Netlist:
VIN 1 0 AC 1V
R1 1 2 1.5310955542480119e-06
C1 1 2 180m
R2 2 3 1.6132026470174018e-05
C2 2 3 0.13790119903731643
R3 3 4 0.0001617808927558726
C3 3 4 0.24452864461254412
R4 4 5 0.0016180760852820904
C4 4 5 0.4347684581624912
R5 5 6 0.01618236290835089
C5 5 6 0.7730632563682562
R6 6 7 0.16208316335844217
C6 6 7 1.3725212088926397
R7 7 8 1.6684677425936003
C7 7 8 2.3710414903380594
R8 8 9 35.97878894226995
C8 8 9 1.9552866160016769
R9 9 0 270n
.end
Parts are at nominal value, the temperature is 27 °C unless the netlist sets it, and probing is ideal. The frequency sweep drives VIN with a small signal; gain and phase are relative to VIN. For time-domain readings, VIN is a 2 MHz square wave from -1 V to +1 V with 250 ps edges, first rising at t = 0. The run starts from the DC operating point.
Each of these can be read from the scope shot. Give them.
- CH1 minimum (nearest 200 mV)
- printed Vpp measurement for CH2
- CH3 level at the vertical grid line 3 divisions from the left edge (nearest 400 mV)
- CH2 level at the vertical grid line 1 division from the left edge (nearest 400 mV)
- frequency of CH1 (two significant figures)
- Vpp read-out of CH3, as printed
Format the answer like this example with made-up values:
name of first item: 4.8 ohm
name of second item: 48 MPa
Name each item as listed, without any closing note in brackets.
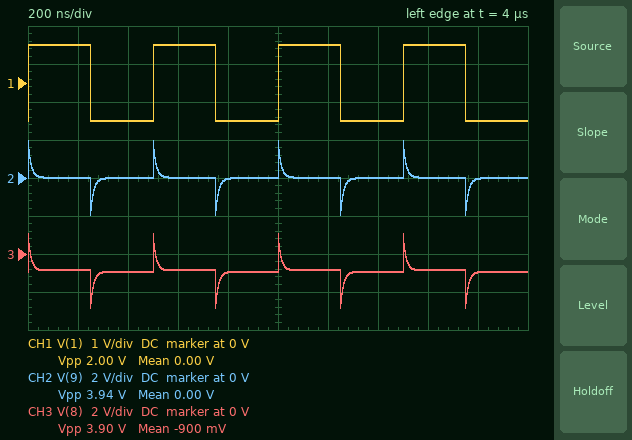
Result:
CH1 minimum: -1.0 V
printed Vpp measurement for CH2: 3.94 V
CH3 level at the vertical grid line 3 divisions from the left edge: -800 mV
CH2 level at the vertical grid line 1 division from the left edge: 0 V
frequency of CH1: 2.0 MHz
Vpp read-out of CH3, as printed: 3.90 V
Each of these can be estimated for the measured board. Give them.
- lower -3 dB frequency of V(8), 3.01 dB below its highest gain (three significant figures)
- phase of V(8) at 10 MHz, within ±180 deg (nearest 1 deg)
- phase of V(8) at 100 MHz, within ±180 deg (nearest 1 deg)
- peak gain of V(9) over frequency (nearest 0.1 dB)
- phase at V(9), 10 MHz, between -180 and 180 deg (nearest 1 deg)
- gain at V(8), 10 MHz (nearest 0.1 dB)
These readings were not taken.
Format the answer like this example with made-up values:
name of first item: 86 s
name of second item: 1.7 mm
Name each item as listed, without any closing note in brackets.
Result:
lower -3 dB frequency of V(8), 3.01 dB below its highest gain: 13.2 MHz
phase of V(8) at 10 MHz, within ±180 deg: 50 deg
phase of V(8) at 100 MHz, within ±180 deg: 7 deg
peak gain of V(9) over frequency: 0 dB
phase at V(9), 10 MHz, between -180 and 180 deg: 52 deg
gain at V(8), 10 MHz: -4.4 dB
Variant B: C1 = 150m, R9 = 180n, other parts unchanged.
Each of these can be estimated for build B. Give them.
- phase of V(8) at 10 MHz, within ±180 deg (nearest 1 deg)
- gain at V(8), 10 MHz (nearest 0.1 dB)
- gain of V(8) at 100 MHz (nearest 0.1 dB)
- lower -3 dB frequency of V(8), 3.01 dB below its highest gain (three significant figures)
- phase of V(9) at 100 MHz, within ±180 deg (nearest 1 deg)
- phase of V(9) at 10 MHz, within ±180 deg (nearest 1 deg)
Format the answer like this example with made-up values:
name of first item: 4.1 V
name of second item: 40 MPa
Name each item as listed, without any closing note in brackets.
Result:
phase of V(8) at 10 MHz, within ±180 deg: 60 deg
gain at V(8), 10 MHz: -7.2 dB
gain of V(8) at 100 MHz: -0.2 dB
lower -3 dB frequency of V(8), 3.01 dB below its highest gain: 20.8 MHz
phase of V(9) at 100 MHz, within ±180 deg: 12 deg
phase of V(9) at 10 MHz, within ±180 deg: 63 deg
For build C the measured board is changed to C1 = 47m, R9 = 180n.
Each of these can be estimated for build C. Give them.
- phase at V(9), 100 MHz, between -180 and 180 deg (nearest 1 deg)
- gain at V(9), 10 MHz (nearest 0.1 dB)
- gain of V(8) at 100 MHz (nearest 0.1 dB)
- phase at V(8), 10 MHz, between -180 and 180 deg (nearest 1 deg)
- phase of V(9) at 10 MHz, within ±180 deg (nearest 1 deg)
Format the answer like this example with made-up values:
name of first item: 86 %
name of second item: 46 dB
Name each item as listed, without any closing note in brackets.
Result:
phase at V(9), 100 MHz, between -180 and 180 deg: 18 deg
gain at V(9), 10 MHz: -11.0 dB
gain of V(8) at 100 MHz: -0.5 dB
phase at V(8), 10 MHz, between -180 and 180 deg: 64 deg
phase of V(9) at 10 MHz, within ±180 deg: 67 deg
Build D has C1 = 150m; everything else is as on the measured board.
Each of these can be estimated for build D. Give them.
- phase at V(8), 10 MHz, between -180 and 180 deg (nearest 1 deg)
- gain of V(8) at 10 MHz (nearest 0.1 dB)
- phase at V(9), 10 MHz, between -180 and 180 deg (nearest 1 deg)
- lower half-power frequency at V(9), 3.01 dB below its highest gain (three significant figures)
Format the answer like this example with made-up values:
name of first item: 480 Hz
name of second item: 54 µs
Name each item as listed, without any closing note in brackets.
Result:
phase at V(8), 10 MHz, between -180 and 180 deg: 51 deg
gain of V(8) at 10 MHz: -4.7 dB
phase at V(9), 10 MHz, between -180 and 180 deg: 53 deg
lower half-power frequency at V(9), 3.01 dB below its highest gain: 13.9 MHz
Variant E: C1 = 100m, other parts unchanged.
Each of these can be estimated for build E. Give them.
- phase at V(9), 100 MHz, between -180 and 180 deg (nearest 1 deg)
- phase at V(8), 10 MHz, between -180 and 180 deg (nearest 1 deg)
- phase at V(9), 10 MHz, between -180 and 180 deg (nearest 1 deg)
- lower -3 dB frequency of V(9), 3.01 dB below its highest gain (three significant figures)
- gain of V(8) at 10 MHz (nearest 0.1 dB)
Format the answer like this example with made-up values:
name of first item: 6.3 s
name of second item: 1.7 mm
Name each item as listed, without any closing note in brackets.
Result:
phase at V(9), 100 MHz, between -180 and 180 deg: 9 deg
phase at V(8), 10 MHz, between -180 and 180 deg: 54 deg
phase at V(9), 10 MHz, between -180 and 180 deg: 56 deg
lower -3 dB frequency of V(9), 3.01 dB below its highest gain: 16.1 MHz
gain of V(8) at 10 MHz: -5.5 dB
